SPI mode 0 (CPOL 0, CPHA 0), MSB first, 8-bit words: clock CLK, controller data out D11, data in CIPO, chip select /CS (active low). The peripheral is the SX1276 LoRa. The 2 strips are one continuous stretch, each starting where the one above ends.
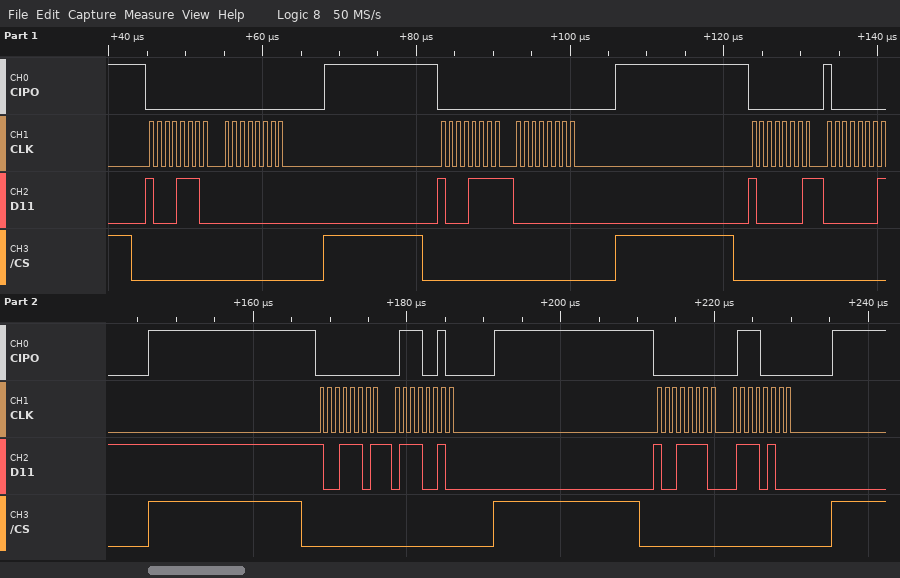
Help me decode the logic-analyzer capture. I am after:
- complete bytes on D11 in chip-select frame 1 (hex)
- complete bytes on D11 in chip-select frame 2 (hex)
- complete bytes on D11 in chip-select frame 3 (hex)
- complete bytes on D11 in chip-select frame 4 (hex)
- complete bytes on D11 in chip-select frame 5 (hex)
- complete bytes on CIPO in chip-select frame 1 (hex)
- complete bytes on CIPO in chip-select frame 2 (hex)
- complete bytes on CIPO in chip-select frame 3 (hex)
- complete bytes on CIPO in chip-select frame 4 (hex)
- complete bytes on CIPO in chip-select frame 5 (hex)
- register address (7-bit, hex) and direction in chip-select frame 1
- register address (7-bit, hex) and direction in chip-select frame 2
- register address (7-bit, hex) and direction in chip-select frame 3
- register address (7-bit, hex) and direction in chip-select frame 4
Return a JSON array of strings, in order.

["0x8E 0x00", "0x8F 0x00", "0x81 0x01", "0x9D 0x72", "0x9E 0x74", "0x00 0x00", "0x00 0x00", "0x00 0x80", "0x00 0x72", "0x00 0x70", "0x0E write", "0x0F write", "0x01 write", "0x1D write"]
